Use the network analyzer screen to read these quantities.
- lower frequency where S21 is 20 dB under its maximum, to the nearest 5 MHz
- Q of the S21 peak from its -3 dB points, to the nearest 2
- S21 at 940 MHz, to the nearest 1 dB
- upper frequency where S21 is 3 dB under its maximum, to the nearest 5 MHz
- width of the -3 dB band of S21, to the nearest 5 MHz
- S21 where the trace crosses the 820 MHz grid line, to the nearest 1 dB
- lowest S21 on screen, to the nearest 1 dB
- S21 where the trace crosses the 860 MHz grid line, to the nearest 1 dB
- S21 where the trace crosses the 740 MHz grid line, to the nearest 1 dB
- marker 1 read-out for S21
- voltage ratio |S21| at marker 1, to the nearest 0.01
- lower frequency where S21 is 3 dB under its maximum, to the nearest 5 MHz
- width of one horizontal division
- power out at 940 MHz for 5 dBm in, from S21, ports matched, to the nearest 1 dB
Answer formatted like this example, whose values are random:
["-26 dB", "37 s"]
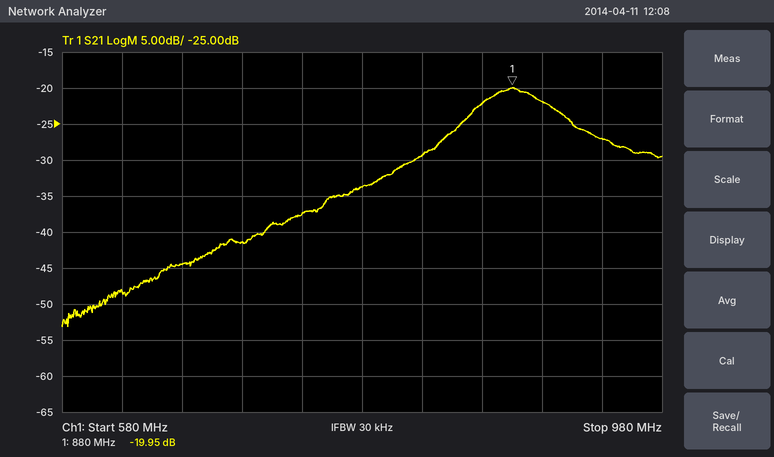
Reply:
["715 MHz", "16", "-27 dB", "910 MHz", "55 MHz", "-29 dB", "-53 dB", "-22 dB", "-37 dB", "-19.95 dB", "0.10", "855 MHz", "40 MHz", "-22 dBm"]
